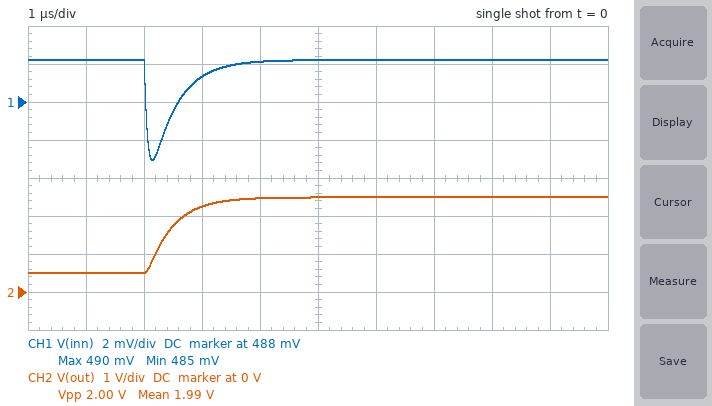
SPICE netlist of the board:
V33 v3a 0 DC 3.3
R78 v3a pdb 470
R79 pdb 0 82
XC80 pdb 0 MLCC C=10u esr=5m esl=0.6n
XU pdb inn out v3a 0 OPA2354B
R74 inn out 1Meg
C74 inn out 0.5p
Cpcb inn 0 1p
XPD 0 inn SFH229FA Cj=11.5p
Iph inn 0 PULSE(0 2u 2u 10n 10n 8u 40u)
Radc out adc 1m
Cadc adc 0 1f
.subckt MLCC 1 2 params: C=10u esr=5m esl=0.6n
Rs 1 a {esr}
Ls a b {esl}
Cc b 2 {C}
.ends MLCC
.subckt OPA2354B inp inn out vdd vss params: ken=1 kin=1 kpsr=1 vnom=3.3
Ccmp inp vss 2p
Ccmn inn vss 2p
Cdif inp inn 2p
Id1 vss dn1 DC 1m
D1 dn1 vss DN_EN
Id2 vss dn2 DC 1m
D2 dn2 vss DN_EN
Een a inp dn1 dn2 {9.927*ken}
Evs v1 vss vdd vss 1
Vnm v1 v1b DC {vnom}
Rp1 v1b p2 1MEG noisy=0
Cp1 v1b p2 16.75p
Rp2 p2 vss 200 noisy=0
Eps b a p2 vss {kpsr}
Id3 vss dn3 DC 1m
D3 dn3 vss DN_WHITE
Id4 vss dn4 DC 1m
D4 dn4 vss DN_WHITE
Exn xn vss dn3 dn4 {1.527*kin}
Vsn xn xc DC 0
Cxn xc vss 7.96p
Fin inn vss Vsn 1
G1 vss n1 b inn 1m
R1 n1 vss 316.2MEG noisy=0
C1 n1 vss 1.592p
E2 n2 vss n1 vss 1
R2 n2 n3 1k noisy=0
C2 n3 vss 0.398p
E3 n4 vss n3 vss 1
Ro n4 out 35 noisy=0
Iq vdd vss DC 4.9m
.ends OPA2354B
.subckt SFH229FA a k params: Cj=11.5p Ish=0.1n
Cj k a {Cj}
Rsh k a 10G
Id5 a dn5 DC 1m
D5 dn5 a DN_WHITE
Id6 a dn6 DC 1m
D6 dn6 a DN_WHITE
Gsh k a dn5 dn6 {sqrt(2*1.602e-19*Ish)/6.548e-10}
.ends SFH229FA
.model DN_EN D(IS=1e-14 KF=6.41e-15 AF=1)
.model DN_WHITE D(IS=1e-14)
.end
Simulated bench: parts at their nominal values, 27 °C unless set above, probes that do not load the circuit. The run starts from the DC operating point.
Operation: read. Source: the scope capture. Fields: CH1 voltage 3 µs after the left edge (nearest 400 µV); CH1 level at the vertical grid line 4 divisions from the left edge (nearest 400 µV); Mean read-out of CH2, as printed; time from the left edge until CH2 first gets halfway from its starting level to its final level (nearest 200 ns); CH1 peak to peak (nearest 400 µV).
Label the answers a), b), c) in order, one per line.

a) 489.2 mV
b) 490.0 mV
c) 1.99 V
d) 2.4 µs
e) 5.2 mV
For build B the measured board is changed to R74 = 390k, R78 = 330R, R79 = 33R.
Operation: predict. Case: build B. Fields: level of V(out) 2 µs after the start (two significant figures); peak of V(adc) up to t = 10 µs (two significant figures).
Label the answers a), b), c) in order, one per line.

a) 300 mV
b) 1.1 V
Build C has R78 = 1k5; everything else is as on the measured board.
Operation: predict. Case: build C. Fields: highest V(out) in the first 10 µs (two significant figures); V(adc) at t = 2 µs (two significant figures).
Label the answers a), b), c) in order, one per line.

a) 2.2 V
b) 170 mV
